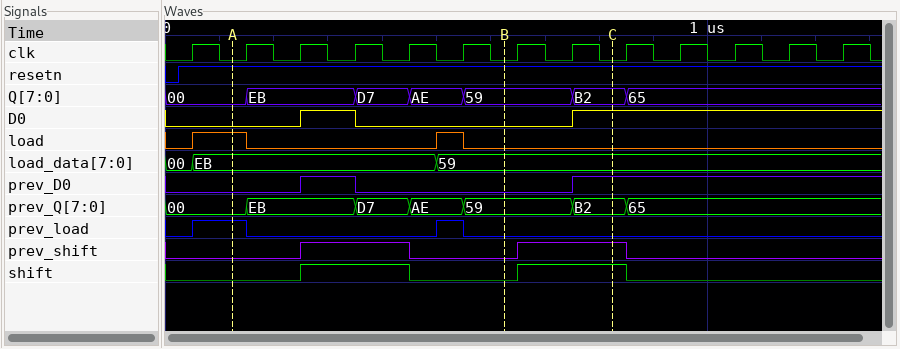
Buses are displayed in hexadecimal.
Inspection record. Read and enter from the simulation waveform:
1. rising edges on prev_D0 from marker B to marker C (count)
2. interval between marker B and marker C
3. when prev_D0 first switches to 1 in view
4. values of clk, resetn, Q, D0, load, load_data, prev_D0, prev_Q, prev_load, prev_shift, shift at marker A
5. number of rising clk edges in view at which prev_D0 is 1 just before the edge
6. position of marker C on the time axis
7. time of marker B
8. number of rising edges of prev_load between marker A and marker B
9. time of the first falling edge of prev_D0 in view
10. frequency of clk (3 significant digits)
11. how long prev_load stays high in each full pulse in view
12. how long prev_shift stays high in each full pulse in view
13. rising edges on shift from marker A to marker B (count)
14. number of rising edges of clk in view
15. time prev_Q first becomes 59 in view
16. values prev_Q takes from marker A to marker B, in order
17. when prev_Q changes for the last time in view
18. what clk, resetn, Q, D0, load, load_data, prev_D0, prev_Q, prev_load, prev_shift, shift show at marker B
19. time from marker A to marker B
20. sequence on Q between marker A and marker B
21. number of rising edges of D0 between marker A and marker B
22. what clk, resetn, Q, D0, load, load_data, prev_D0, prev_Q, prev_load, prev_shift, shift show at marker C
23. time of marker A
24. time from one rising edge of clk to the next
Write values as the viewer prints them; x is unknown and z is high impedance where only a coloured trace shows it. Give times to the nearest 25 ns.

1
200 ns
250 ns
clk=0, resetn=1, Q=00, D0=0, load=1, load_data=EB, prev_D0=0, prev_Q=00, prev_load=1, prev_shift=0, shift=0
6
825 ns
625 ns
1
350 ns
10.0 MHz
100 ns, 50 ns
200 ns, 200 ns
1
13
550 ns
00, EB, D7, AE, 59
850 ns
clk=0, resetn=1, Q=59, D0=0, load=0, load_data=59, prev_D0=0, prev_Q=59, prev_load=0, prev_shift=0, shift=0
500 ns
00, EB, D7, AE, 59
1
clk=0, resetn=1, Q=B2, D0=1, load=0, load_data=59, prev_D0=1, prev_Q=B2, prev_load=0, prev_shift=1, shift=1
125 ns
100 ns
